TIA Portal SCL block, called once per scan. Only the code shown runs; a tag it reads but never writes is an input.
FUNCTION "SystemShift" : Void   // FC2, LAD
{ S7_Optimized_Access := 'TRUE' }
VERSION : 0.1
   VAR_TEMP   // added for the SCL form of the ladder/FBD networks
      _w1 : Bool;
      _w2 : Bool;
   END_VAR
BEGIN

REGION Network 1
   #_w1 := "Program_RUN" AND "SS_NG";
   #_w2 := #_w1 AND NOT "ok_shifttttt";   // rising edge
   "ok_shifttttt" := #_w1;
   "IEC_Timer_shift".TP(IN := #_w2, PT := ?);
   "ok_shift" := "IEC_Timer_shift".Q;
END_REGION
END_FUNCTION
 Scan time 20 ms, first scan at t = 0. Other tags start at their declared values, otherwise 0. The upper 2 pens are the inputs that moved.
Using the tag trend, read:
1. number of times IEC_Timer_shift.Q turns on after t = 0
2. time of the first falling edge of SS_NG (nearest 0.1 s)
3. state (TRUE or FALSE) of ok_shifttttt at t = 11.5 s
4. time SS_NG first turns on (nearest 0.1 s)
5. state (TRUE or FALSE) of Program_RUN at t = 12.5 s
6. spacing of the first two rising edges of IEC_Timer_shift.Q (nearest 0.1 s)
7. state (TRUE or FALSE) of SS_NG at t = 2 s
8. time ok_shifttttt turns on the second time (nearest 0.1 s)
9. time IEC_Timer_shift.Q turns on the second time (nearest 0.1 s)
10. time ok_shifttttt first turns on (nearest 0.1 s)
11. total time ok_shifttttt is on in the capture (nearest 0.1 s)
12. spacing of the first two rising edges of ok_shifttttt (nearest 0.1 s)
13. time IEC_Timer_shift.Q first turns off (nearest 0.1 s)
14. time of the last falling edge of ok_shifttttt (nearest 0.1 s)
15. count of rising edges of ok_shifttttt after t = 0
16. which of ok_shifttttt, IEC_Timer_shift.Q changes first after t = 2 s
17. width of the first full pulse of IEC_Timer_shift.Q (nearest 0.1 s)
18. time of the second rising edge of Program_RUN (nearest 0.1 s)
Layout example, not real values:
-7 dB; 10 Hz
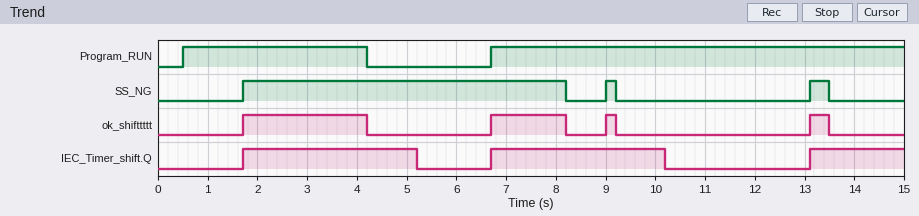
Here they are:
3; 8.2 s; FALSE; 1.7 s; TRUE; 5.0 s; TRUE; 6.7 s; 6.7 s; 1.7 s; 4.6 s; 5.0 s; 5.2 s; 13.5 s; 4; ok_shifttttt; 3.5 s; 6.7 s
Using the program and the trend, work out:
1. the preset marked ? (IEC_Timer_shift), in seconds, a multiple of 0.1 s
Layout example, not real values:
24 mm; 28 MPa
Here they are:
3.5 s
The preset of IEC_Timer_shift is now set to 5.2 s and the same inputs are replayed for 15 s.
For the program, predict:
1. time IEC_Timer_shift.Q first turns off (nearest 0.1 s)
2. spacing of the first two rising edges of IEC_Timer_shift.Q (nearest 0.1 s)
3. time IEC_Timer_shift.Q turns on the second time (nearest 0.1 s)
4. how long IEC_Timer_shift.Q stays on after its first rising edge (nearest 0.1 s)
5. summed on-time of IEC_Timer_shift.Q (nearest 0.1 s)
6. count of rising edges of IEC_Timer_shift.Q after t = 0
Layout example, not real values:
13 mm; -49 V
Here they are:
6.9 s; 7.3 s; 9.0 s; 5.2 s; 10.4 s; 2
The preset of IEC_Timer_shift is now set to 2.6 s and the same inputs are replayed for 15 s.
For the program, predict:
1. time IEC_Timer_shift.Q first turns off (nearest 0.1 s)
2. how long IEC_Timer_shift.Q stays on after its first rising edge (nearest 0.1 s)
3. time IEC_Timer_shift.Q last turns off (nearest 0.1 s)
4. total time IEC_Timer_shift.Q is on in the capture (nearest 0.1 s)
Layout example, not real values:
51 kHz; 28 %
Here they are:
4.3 s; 2.6 s; 9.3 s; 7.1 s
